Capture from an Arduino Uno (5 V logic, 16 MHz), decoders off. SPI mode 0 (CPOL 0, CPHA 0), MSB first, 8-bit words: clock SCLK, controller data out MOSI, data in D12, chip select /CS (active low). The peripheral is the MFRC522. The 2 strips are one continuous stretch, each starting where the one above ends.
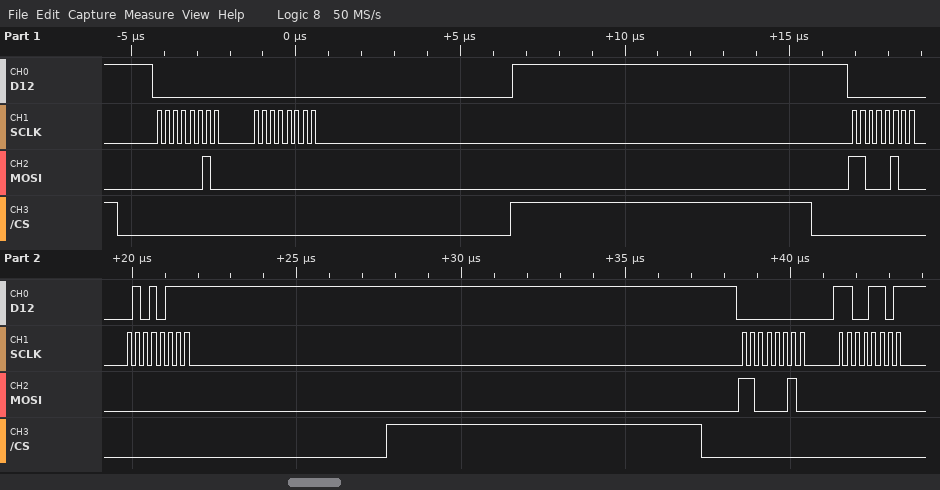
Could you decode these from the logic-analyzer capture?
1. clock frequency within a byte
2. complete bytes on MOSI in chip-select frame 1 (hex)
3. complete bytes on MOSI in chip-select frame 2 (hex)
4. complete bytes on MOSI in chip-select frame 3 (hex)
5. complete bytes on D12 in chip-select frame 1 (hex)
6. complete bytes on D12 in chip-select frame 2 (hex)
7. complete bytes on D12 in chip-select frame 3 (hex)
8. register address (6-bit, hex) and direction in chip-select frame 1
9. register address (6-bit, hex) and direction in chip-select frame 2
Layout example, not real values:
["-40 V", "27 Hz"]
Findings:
["4 MHz", "02 00", "C4 00", "C2 00", "00 00", "00 57", "00 CD", "0x01 write", "0x22 read"]
